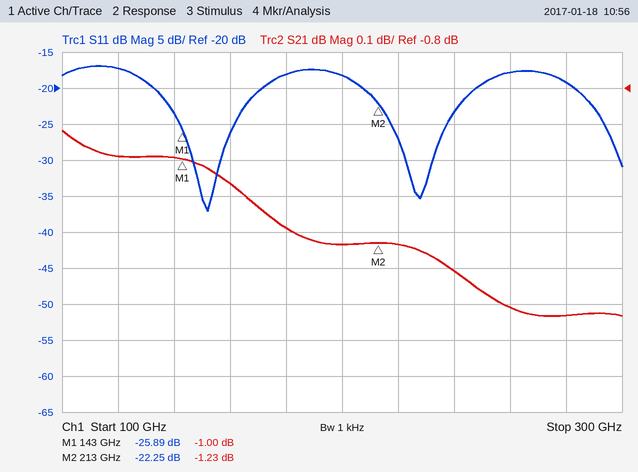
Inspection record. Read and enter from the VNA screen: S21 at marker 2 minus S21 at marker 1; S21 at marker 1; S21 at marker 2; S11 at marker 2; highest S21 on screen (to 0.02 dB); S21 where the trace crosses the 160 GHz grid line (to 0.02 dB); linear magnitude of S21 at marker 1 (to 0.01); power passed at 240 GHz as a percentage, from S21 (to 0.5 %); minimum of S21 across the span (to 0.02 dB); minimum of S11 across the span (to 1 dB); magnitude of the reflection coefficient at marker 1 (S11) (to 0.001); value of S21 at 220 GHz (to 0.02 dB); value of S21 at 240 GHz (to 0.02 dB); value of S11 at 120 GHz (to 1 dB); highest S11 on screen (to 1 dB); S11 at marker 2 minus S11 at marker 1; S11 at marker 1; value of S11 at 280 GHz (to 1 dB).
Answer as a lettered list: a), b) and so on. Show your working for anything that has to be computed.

a) -1.23 − (-1) = -0.23 dB
b) -1.00 dB
c) -1.23 dB
d) -22.25 dB
e) -0.92 dB
f) -1.06 dB
g) 10^(-1/20) ≈ 0.89
h) 10^(-1.3/10) ≈ 74.1 %, so 74.0 % to the nearest 0.5 %
i) -1.44 dB
j) -37 dB
k) 10^(-25.89/20) ≈ 0.051
l) -1.24 dB
m) -1.30 dB
n) -17 dB
o) -17 dB
p) -22.25 − (-25.89) = 3.64 dB
q) -25.89 dB
r) -19 dB
